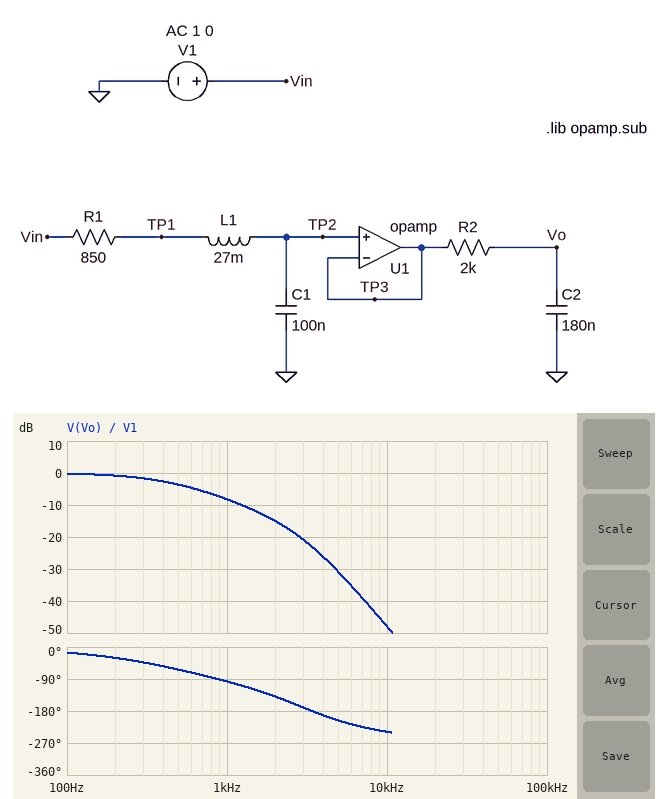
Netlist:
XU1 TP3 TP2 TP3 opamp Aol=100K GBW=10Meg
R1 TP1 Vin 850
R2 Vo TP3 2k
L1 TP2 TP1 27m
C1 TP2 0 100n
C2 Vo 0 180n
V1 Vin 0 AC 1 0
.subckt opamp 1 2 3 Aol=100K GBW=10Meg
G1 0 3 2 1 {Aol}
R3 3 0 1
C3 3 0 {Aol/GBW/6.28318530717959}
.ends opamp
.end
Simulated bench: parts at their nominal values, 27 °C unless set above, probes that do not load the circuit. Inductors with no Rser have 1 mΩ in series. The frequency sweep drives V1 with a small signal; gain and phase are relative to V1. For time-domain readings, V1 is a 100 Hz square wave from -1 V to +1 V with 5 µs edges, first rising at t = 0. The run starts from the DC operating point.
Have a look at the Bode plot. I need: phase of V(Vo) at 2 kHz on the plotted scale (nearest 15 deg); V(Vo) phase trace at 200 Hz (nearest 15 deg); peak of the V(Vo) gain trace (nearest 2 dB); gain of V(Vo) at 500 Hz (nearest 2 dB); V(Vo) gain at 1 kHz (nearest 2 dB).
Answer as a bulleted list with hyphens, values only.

- -135 deg
- -30 deg
- 0 dB
- -4 dB
- -8 dB
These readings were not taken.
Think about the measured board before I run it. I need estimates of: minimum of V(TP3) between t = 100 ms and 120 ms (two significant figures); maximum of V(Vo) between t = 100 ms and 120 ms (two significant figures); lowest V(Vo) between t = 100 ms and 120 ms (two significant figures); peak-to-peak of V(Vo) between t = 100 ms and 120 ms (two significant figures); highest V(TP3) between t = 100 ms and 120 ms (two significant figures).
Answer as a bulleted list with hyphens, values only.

- -1.0 V
- 1.0 V
- -1.0 V
- 2.0 V
- 1.0 V
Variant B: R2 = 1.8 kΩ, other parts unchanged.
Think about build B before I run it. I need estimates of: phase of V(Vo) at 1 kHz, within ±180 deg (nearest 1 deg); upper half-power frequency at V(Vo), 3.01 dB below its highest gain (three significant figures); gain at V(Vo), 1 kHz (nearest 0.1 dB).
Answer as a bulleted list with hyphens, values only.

- -95 deg
- 483 Hz
- -7.5 dB
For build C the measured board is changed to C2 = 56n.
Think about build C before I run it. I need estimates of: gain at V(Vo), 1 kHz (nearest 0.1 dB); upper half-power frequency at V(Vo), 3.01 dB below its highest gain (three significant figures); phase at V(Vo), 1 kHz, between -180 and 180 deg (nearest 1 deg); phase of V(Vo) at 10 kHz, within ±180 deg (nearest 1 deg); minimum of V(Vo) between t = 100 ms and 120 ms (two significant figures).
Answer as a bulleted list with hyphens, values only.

- -2.1 dB
- 1.24 kHz
- -66 deg
- 127 deg
- -1.0 V
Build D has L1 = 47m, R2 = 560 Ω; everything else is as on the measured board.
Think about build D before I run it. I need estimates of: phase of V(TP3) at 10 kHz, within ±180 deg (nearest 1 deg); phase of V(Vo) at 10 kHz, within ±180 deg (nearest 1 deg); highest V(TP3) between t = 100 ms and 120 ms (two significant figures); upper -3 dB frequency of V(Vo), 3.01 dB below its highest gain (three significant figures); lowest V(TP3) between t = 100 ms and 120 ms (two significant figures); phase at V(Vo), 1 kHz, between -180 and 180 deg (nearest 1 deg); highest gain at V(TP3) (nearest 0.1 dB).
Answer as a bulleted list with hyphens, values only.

- -163 deg
- 116 deg
- 1.2 V
- 1.58 kHz
- -1.2 V
- -66 deg
- 0.2 dB
